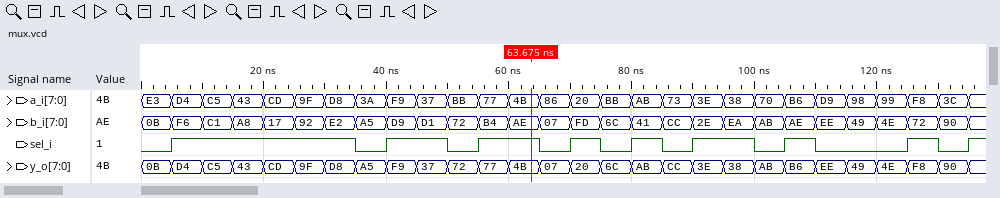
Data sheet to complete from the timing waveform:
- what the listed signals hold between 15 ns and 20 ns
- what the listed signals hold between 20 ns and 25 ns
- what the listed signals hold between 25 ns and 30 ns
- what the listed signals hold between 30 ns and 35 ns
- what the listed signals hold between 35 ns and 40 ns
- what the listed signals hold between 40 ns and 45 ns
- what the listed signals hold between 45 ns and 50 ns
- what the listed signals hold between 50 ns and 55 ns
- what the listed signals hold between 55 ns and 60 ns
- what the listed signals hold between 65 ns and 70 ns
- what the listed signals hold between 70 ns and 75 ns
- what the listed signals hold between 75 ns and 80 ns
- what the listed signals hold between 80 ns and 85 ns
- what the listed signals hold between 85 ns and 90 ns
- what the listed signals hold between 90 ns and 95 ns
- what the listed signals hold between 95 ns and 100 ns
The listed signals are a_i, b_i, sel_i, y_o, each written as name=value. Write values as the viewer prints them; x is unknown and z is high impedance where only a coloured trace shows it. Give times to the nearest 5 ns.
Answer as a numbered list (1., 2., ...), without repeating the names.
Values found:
1. a_i=43, b_i=A8, sel_i=1, y_o=43
2. a_i=CD, b_i=17, sel_i=1, y_o=CD
3. a_i=9F, b_i=92, sel_i=1, y_o=9F
4. a_i=D8, b_i=E2, sel_i=1, y_o=D8
5. a_i=3A, b_i=A5, sel_i=0, y_o=A5
6. a_i=F9, b_i=D9, sel_i=1, y_o=F9
7. a_i=37, b_i=D1, sel_i=1, y_o=37
8. a_i=BB, b_i=72, sel_i=0, y_o=72
9. a_i=77, b_i=B4, sel_i=1, y_o=77
10. a_i=86, b_i=07, sel_i=0, y_o=07
11. a_i=20, b_i=FD, sel_i=1, y_o=20
12. a_i=BB, b_i=6C, sel_i=0, y_o=6C
13. a_i=AB, b_i=41, sel_i=1, y_o=AB
14. a_i=73, b_i=CC, sel_i=0, y_o=CC
15. a_i=3E, b_i=2E, sel_i=1, y_o=3E
16. a_i=38, b_i=EA, sel_i=1, y_o=38
